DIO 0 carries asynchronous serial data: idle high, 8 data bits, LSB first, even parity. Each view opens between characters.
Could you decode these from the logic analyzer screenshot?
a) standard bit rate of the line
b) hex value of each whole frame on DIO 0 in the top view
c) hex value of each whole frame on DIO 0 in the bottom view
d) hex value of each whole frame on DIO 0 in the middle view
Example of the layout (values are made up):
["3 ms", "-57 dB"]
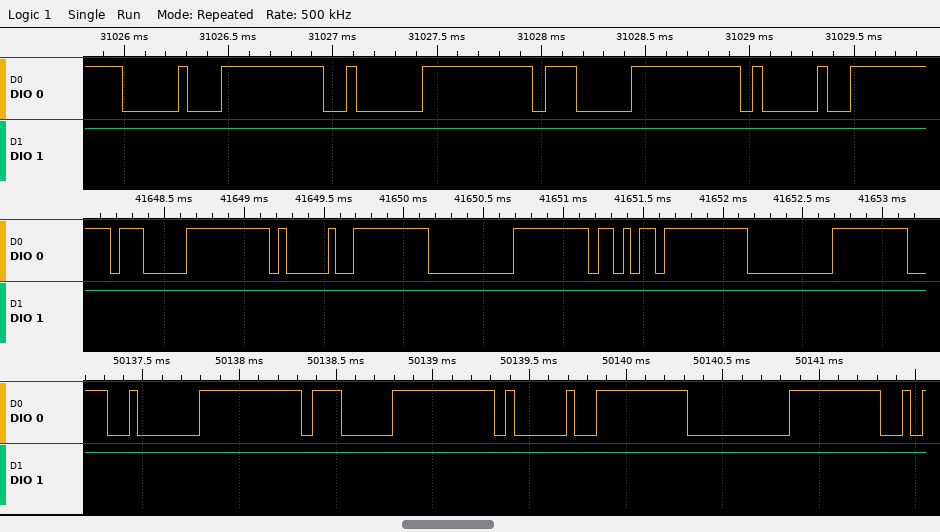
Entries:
["19200 baud", "10, 02, 07, 41", "02, 07, 41, 00", "07, 41, 00, 6B, 00"]
